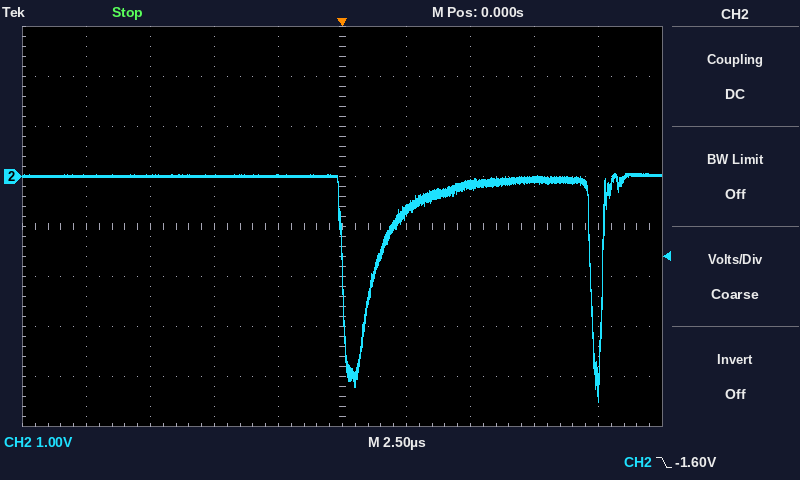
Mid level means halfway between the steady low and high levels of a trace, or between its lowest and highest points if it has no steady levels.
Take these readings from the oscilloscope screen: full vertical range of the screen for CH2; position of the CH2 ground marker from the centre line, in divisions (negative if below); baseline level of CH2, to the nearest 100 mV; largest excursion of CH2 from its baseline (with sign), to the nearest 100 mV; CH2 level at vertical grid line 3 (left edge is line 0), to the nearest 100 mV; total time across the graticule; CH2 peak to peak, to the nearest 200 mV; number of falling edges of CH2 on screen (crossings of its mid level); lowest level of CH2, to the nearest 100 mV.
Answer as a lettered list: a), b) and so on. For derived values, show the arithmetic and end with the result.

a) 8 V
b) +1.0 div
c) 0.0 V
d) -4.5 V − (0.0 V) = -4.5 V
e) 0.0 V
f) 25 µs
g) 4.6 V
h) 2
i) -4.5 V
